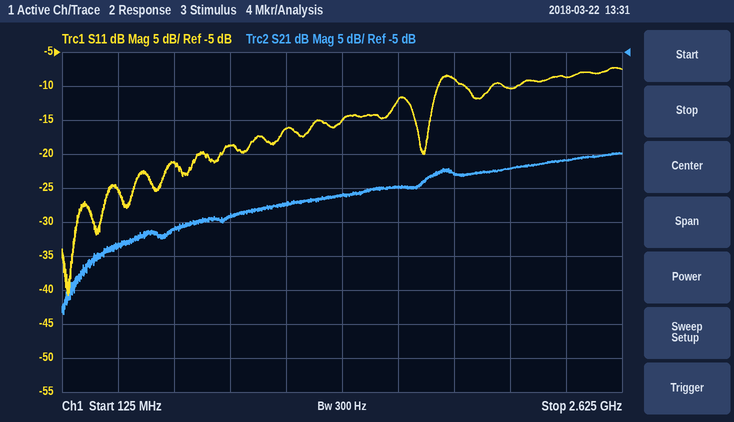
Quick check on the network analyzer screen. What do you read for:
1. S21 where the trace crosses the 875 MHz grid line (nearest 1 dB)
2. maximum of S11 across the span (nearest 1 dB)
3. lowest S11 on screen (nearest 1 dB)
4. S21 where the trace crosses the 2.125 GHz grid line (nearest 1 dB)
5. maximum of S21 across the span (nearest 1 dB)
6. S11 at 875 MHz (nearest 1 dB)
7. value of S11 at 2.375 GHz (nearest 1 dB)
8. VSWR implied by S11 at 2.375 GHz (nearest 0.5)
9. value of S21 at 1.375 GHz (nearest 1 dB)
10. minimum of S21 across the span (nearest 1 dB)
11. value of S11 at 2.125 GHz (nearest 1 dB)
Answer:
-29 dB
-7 dB
-41 dB
-22 dB
-20 dB
-19 dB
-9 dB
2.0
-26 dB
-44 dB
-10 dB
